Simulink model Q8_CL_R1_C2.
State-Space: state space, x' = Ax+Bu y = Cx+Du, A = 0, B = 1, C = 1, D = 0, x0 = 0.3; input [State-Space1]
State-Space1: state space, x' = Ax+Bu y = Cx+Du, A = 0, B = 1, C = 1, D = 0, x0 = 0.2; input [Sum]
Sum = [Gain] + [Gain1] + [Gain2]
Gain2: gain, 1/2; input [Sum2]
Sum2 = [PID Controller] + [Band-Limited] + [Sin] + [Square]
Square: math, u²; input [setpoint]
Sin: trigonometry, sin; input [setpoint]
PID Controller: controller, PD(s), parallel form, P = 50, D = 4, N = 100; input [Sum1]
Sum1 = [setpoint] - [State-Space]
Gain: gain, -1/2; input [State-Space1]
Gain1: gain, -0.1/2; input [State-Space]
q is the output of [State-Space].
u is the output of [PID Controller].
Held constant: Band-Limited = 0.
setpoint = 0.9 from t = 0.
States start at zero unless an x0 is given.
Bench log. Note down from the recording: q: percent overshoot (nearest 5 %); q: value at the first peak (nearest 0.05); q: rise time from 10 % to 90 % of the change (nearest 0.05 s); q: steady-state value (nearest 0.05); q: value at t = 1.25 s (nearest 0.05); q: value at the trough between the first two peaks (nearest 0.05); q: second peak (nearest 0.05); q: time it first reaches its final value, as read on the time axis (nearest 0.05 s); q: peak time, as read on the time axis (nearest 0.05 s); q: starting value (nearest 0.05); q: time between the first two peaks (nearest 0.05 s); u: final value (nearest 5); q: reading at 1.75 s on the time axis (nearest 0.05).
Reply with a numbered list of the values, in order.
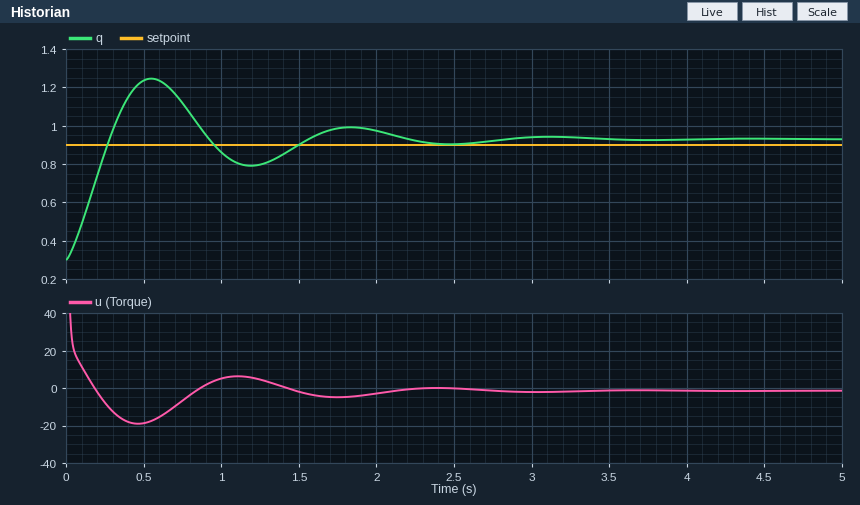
1. 50 %
2. 1.25
3. 0.20 s
4. 0.95
5. 0.80
6. 0.80
7. 1.00
8. 0.30 s
9. 0.55 s
10. 0.30
11. 1.30 s
12. 0
13. 1.00
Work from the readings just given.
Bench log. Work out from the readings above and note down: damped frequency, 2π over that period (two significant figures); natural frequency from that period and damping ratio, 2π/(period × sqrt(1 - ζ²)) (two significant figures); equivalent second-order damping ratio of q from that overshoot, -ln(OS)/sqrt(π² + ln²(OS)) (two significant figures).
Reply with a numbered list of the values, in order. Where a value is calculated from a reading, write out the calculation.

1. 2π / 1.3 = 4.8 rad/s
2. 2π / (1.3 × sqrt(1 - 0.22²)) = 5.0 rad/s
3. ln(0.5) = -0.693; 0.693 / sqrt(9.870 + 0.480) = 0.22
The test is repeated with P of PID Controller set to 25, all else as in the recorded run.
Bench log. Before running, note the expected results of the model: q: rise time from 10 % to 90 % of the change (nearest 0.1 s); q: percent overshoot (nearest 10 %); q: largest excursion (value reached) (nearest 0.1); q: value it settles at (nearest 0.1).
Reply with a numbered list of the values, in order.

1. 0.3 s
2. 40 %
3. 1.2
4. 1.0
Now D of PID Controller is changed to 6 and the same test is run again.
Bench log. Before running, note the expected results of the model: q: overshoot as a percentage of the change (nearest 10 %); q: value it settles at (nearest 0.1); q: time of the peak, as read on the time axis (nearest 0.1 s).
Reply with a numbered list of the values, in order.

1. 40 %
2. 0.9
3. 0.5 s
